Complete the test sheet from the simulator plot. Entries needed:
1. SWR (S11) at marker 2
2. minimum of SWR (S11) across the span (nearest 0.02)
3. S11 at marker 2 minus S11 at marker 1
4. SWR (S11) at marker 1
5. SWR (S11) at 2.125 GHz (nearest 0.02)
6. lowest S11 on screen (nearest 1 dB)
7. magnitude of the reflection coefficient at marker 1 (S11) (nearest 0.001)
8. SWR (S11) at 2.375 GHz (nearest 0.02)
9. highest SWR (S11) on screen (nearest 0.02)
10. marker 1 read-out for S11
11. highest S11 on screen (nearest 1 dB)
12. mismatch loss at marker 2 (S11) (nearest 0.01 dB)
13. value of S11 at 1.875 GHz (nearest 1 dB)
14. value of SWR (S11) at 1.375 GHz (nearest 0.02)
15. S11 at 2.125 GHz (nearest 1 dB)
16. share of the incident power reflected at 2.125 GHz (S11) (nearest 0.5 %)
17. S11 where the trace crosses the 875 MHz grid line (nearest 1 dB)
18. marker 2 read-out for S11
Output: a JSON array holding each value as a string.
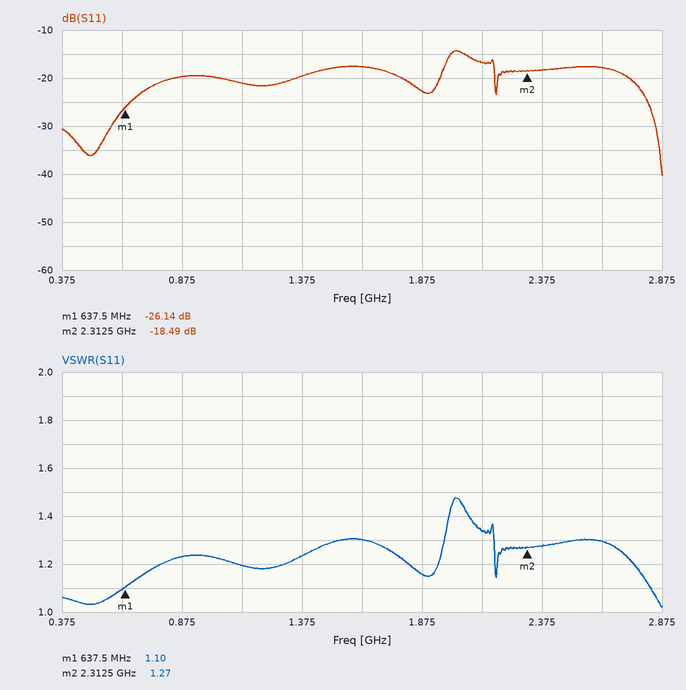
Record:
["1.27", "1.02", "7.65 dB", "1.10", "1.34", "-40 dB", "0.049", "1.28", "1.48", "-26.14 dB", "-14 dB", "0.06 dB", "-23 dB", "1.24", "-17 dB", "2.0 %", "-20 dB", "-18.49 dB"]
